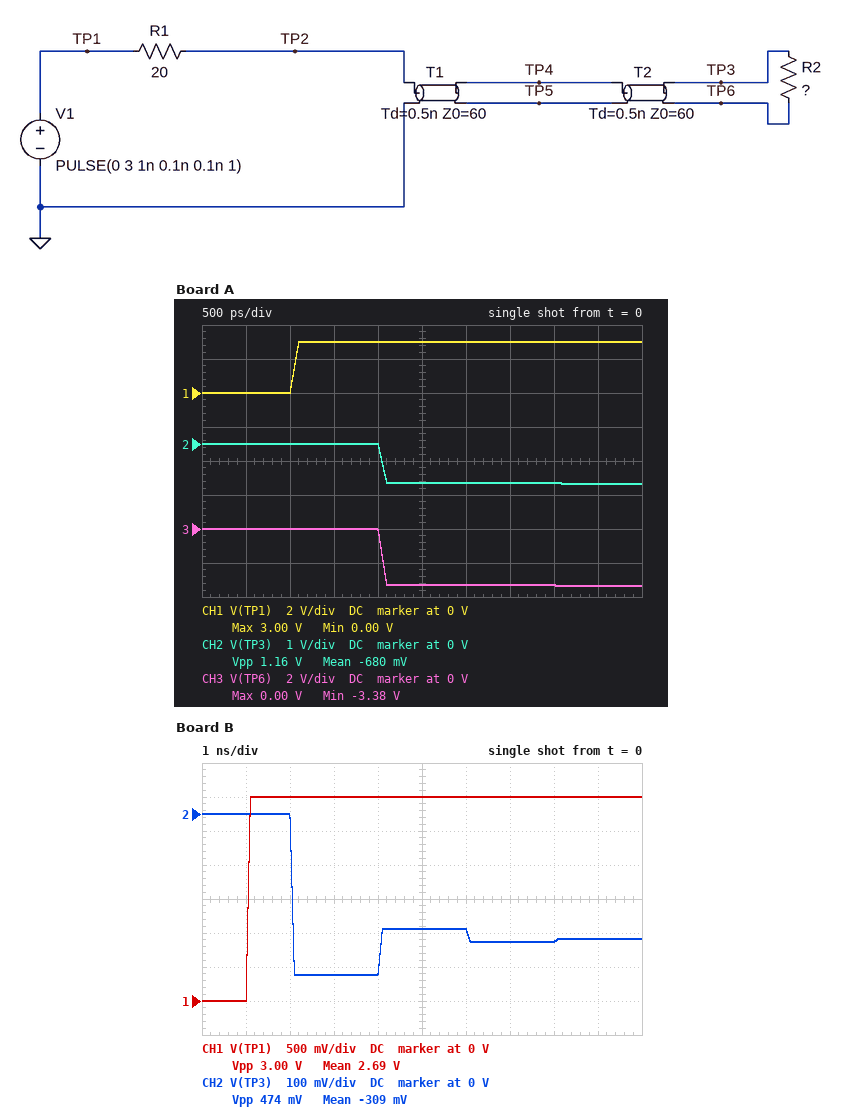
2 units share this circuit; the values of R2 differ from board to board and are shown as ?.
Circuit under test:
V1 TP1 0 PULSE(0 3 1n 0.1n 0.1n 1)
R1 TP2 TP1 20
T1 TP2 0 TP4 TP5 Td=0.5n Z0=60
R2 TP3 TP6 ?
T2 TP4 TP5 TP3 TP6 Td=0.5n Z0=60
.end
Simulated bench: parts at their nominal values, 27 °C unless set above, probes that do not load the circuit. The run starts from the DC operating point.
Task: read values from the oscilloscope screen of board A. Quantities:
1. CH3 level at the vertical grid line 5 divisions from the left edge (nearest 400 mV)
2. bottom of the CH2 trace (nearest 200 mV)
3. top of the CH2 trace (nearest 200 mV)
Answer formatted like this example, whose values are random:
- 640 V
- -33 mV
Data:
- -3.2 V
- -1.2 V
- 0 V
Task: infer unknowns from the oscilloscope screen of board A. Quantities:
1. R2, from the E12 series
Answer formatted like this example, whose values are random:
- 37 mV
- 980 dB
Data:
- 56 Ω
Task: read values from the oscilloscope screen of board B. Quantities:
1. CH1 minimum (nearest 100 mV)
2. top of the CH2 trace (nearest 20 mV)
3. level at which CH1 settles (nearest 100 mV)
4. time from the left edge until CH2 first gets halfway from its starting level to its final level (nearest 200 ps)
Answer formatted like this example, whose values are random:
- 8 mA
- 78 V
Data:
- 0 V
- 0 V
- 3.0 V
- 2.0 ns
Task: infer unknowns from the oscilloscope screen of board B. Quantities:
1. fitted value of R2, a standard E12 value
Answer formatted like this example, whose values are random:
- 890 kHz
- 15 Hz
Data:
- 220 Ω
